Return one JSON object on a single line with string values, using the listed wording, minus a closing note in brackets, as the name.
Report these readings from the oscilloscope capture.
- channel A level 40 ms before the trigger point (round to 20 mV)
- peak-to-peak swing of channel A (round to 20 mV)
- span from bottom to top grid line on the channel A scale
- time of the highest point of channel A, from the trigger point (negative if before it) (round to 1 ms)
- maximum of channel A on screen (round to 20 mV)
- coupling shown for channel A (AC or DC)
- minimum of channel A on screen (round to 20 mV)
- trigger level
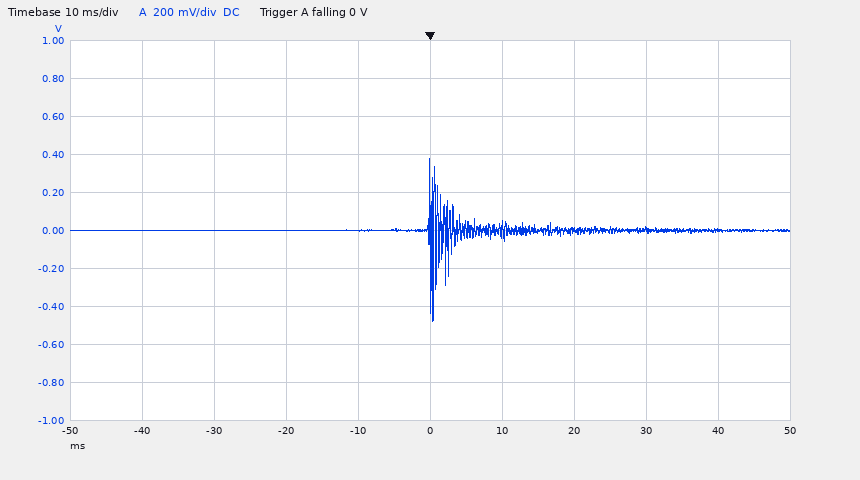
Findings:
{"channel A level 40 ms before the trigger point": "0 mV", "peak-to-peak swing of channel A": "860 mV", "span from bottom to top grid line on the channel A scale": "2 V", "time of the highest point of channel A, from the trigger point (negative if before it)": "0 ms", "maximum of channel A on screen": "380 mV", "coupling shown for channel A": "DC", "minimum of channel A on screen": "-480 mV", "trigger level": "0 V"}
